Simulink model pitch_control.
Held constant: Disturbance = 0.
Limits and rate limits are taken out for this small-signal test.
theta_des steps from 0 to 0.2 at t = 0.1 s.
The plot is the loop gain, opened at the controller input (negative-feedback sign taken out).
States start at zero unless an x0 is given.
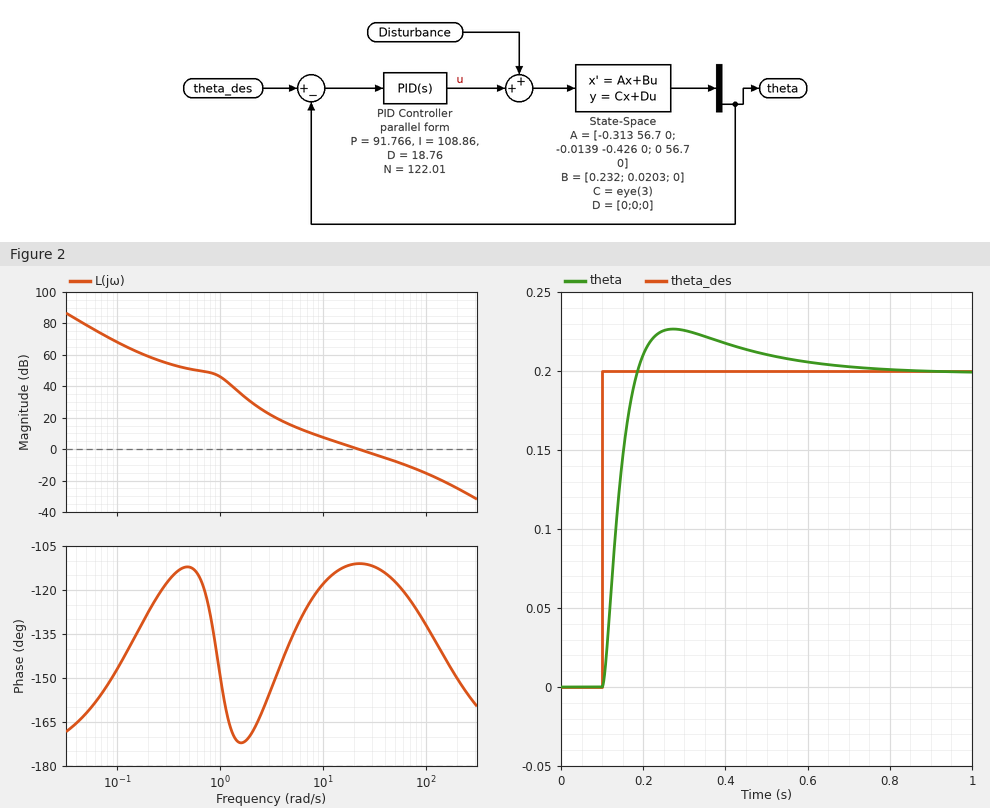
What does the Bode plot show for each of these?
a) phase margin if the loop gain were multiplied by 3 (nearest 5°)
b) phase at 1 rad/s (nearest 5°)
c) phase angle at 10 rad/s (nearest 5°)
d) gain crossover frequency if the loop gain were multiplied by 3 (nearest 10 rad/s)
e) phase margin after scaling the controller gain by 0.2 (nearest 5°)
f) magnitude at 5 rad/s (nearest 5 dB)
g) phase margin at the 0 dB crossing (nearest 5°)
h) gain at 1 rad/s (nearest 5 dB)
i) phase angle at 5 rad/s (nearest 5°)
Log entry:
60°
-150°
-120°
60 rad/s
45°
15 dB
70°
45 dB
-135°
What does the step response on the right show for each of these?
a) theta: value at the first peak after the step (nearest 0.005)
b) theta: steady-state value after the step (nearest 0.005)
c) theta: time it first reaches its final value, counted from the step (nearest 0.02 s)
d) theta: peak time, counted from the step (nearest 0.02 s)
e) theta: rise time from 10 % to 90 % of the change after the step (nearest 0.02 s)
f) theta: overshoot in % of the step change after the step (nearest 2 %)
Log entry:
0.225
0.200
0.08 s
0.18 s
0.06 s
14 %
